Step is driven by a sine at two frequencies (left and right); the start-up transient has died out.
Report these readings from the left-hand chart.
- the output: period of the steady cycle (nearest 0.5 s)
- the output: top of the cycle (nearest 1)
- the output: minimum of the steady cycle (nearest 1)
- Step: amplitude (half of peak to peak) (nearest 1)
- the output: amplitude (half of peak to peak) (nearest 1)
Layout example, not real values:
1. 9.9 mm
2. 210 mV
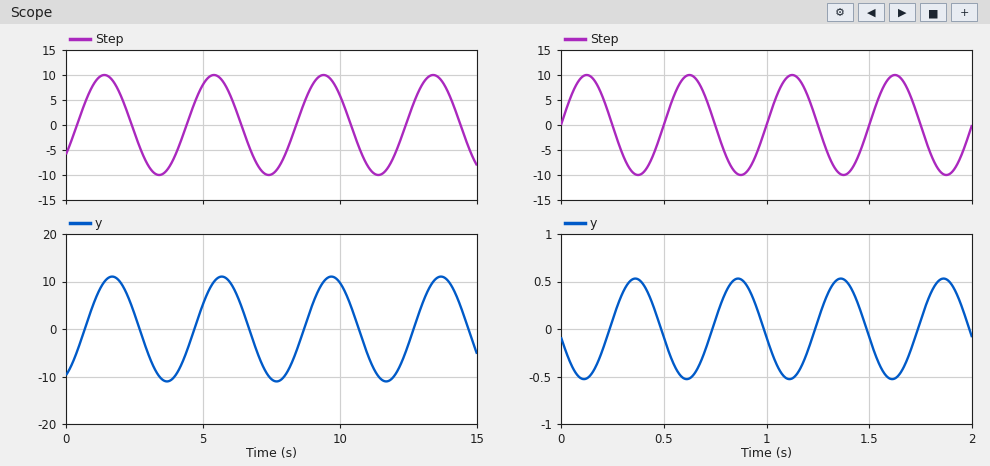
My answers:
1. 4.0 s
2. 11
3. -11
4. 10
5. 11
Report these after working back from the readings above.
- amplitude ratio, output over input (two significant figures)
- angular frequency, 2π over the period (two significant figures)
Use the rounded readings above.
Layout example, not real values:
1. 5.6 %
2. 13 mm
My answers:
1. 1.1
2. 1.6 rad/s
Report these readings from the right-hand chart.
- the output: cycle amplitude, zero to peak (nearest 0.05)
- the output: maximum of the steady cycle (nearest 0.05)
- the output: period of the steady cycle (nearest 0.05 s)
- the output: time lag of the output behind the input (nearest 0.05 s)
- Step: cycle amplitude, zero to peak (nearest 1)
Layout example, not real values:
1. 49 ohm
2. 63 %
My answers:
1. 0.55
2. 0.55
3. 0.50 s
4. 0.25 s
5. 10
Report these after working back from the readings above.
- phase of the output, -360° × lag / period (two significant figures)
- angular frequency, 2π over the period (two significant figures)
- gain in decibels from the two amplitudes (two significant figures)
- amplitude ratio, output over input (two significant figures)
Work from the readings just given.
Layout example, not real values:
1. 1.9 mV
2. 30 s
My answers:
1. -180°
2. 13 rad/s
3. -25 dB
4. 0.055
